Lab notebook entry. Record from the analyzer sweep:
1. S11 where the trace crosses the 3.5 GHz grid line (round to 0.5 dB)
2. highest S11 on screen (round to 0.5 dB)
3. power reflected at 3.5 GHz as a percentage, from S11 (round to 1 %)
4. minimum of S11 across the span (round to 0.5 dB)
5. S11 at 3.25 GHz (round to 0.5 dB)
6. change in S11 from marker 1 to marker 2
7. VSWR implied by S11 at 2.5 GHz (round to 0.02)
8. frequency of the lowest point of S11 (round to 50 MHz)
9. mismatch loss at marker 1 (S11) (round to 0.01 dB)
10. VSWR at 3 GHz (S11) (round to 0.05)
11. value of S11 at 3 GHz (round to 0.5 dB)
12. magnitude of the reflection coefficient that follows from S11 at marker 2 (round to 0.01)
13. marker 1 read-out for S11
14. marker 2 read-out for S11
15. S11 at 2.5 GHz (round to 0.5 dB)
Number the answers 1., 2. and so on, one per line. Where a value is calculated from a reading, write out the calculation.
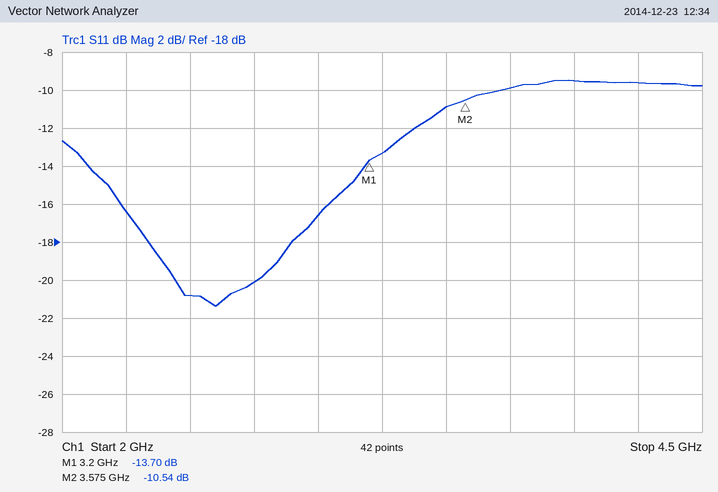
1. -11.0 dB
2. -9.5 dB
3. 10^(-11/10) ≈ 8 %
4. -21.5 dB
5. -13.5 dB
6. -10.54 − (-13.7) = 3.16 dB
7. |Γ| = 10^(-21/20) = 0.0891; VSWR = (1 + 0.0891)/(1 − 0.0891) ≈ 1.20
8. 2.60 GHz
9. −10 log10(1 − 10^(-13.7/10)) ≈ 0.19 dB
10. |Γ| = 10^(-16.5/20) = 0.1496; VSWR = (1 + 0.1496)/(1 − 0.1496) ≈ 1.35
11. -16.5 dB
12. 10^(-10.54/20) ≈ 0.30
13. -13.70 dB
14. -10.54 dB
15. -21.0 dB
